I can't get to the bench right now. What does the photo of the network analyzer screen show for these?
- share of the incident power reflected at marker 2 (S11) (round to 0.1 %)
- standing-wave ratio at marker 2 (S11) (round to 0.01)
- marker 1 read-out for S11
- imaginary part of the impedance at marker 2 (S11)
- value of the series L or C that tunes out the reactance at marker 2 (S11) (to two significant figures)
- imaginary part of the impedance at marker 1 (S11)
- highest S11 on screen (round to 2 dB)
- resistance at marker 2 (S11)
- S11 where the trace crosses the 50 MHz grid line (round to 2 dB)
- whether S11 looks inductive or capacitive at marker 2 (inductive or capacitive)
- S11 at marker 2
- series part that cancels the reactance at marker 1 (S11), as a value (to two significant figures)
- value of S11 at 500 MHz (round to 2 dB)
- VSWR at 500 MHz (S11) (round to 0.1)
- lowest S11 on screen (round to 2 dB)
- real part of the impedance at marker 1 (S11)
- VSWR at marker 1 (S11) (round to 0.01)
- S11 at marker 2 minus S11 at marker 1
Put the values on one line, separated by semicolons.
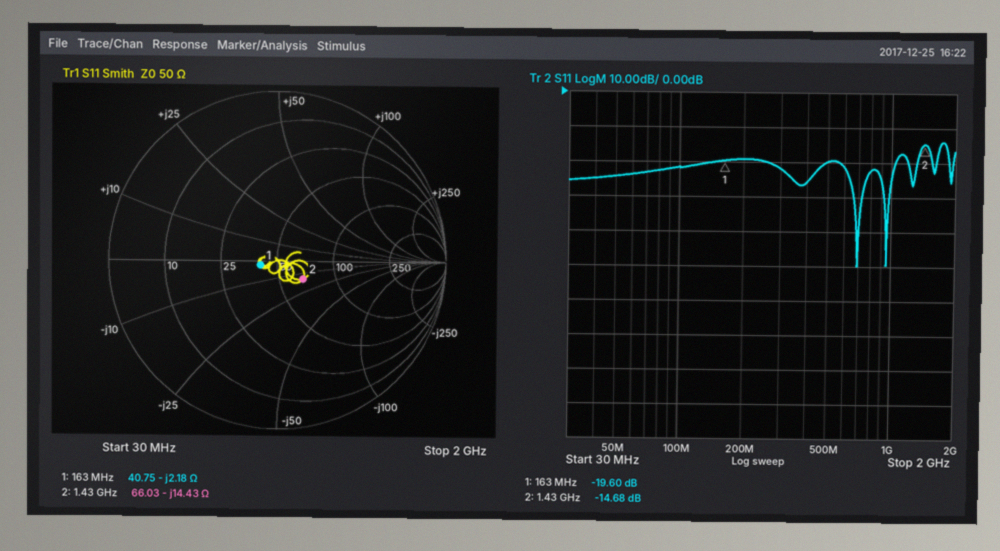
3.4 %; 1.45; -19.60 dB; -14.43 Ω; 1.6 nH; -2.18 Ω; -14 dB; 66.03 Ω; -24 dB; capacitive; -14.68 dB; 2.1 nH; -20 dB; 1.2; -50 dB; 40.75 Ω; 1.23; 4.92 dB
